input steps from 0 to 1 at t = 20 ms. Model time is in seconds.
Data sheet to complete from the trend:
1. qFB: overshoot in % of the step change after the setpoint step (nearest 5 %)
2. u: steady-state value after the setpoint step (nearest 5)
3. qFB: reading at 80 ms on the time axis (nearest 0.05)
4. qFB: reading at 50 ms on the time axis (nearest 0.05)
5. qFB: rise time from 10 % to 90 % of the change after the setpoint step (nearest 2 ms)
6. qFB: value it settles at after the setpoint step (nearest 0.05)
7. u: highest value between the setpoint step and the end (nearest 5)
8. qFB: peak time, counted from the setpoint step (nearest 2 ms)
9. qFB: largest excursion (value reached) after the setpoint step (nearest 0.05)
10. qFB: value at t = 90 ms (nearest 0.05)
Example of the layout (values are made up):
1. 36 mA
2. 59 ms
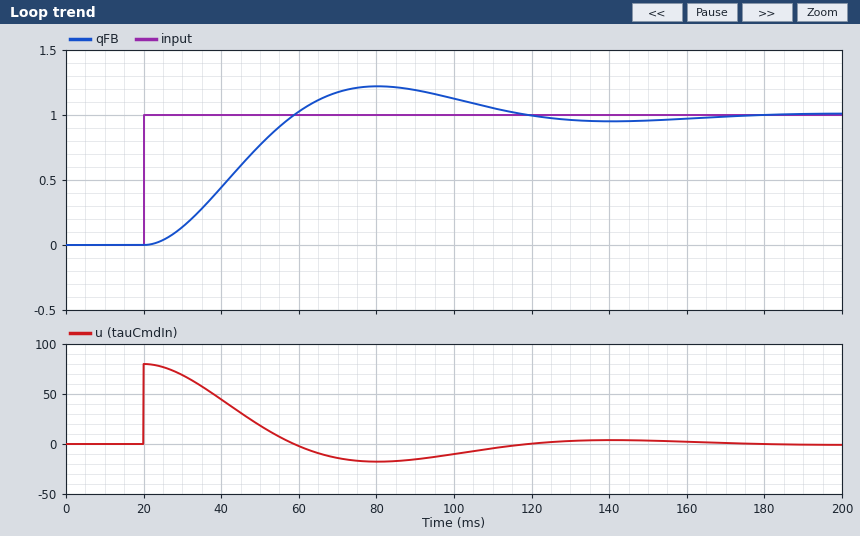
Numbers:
1. 20 %
2. 0
3. 1.20
4. 0.75
5. 26 ms
6. 1.00
7. 80
8. 60 ms
9. 1.20
10. 1.20
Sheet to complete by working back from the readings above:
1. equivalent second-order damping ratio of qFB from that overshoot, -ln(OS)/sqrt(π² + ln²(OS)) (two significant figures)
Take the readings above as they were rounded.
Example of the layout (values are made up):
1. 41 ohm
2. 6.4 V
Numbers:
1. 0.46
